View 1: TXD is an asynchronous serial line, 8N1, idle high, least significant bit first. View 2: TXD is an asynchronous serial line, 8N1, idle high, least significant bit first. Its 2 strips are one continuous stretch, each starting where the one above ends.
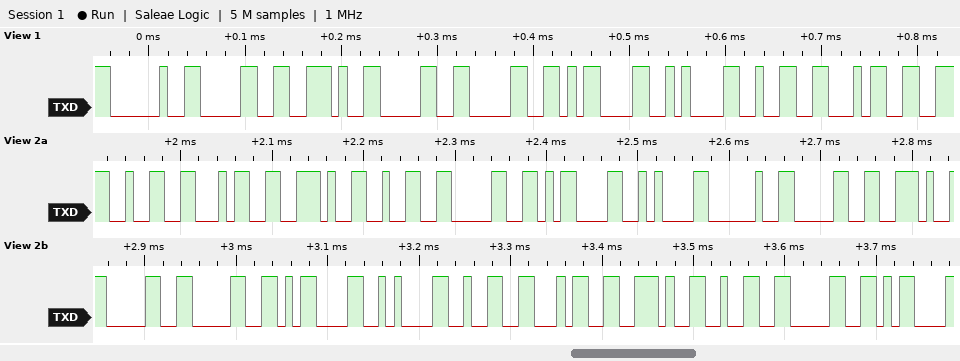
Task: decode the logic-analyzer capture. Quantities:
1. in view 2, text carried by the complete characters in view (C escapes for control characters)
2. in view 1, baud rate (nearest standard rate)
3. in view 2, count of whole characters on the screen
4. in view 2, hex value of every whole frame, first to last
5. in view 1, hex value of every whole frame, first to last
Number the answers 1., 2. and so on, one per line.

1. "24.20\r\n 0.00\r\n24.20\r"
2. 115200 baud
3. 20
4. 0x32 0x34 0x2E 0x32 0x30 0x0D 0x0A 0x20 0x30 0x2E 0x30 0x30 0x0D 0x0A 0x32 0x34 0x2E 0x32 0x30 0x0D
5. 20 30 2E 30 30 0D 0A 32 34
